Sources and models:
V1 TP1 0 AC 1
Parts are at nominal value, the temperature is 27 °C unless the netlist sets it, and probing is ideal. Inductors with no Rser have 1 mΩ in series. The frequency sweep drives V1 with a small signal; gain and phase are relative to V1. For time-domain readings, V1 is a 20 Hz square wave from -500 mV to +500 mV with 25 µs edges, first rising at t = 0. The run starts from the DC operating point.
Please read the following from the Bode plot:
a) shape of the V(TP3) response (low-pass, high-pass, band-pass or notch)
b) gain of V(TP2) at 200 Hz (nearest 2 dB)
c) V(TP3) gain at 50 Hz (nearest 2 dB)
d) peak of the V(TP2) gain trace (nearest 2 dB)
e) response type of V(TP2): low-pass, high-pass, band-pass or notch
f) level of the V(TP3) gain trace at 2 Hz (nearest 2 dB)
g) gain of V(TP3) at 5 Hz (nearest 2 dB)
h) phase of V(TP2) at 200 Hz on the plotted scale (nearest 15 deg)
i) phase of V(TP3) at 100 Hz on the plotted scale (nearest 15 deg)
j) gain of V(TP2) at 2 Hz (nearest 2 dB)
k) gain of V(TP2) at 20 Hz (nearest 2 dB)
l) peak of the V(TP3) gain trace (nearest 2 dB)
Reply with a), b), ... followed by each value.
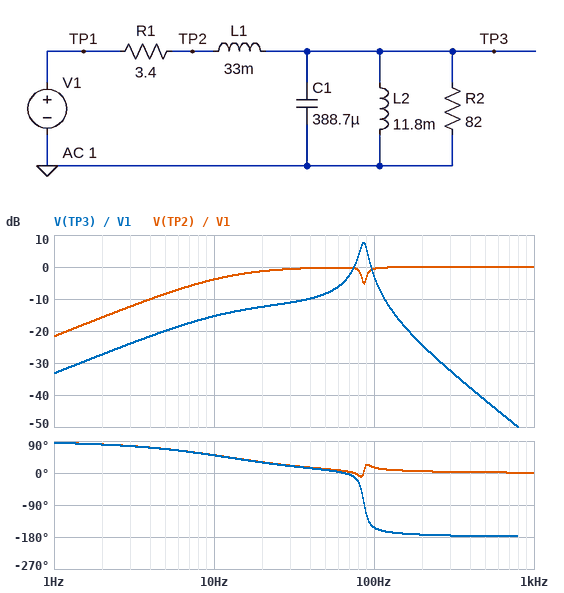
a) band-pass
b) 0 dB
c) -8 dB
d) 0 dB
e) high-pass
f) -28 dB
g) -20 dB
h) 0 deg
i) -150 deg
j) -16 dB
k) -2 dB
l) 8 dB
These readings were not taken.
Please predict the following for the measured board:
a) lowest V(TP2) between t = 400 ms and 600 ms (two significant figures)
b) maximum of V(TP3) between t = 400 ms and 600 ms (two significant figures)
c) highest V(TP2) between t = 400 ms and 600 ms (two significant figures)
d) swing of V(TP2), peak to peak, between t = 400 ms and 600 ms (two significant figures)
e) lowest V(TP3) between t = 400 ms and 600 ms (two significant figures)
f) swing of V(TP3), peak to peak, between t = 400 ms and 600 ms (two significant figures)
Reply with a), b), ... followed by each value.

a) -880 mV
b) 310 mV
c) 880 mV
d) 1.8 V
e) -310 mV
f) 620 mV
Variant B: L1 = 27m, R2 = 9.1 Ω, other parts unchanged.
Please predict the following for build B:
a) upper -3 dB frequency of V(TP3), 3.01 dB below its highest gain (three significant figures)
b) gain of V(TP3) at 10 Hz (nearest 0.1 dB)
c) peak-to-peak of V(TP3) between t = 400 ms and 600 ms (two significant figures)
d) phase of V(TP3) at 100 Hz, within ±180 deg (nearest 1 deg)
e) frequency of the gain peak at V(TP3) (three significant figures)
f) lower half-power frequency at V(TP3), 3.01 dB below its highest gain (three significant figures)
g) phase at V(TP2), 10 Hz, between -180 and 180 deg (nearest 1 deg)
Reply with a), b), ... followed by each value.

a) 106 Hz
b) -15.0 dB
c) 610 mV
d) -102 deg
e) 82.8 Hz
f) 50.6 Hz
g) 53 deg
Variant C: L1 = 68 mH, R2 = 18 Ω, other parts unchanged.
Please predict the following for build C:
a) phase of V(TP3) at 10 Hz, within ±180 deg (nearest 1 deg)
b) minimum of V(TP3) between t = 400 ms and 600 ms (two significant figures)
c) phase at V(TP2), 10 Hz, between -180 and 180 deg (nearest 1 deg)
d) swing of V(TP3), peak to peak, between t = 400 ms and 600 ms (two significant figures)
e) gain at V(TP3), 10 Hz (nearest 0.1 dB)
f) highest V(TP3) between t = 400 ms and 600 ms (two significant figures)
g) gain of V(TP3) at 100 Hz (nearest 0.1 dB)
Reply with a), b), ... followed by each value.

a) 32 deg
b) -170 mV
c) 34 deg
d) 340 mV
e) -18.1 dB
f) 170 mV
g) -12.9 dB
